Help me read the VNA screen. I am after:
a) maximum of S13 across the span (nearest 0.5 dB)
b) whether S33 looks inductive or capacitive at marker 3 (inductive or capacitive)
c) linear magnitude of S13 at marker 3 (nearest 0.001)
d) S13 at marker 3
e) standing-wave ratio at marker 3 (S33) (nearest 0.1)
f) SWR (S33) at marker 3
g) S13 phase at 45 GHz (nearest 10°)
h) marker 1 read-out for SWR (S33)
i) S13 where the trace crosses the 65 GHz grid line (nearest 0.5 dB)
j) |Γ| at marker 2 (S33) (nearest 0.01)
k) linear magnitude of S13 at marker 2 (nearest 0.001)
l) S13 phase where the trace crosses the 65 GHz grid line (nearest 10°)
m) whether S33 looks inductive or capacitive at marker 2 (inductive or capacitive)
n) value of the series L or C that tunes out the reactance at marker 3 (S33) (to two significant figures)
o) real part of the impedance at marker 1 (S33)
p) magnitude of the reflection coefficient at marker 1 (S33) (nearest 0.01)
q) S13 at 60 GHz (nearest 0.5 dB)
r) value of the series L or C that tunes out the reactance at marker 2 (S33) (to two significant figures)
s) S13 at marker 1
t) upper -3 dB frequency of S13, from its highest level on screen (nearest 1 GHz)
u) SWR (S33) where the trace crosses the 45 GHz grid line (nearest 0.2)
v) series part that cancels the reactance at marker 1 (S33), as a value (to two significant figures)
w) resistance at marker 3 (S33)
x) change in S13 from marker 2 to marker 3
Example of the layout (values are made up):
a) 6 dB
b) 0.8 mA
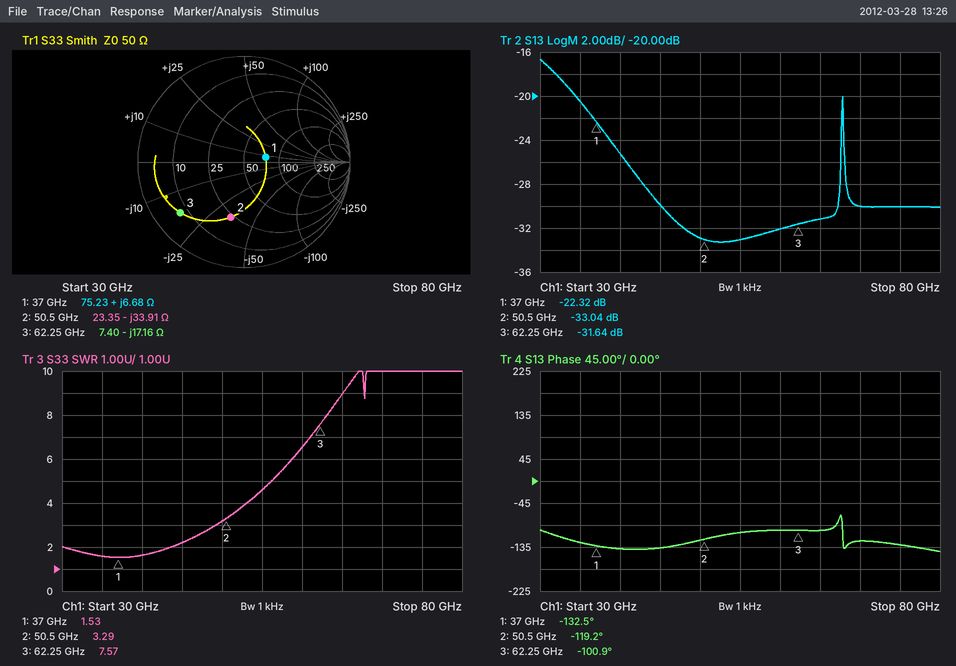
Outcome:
a) -16.5 dB
b) capacitive
c) 0.026
d) -31.64 dB
e) 7.6
f) 7.57
g) -140°
h) 1.53
i) -31.0 dB
j) 0.53
k) 0.022
l) -100°
m) capacitive
n) 44 pH
o) 75.23 Ω
p) 0.21
q) -32.0 dB
r) 110 pH
s) -22.32 dB
t) 34 GHz
u) 2.2
v) 640 fF
w) 7.40 Ω
x) 1.40 dB
